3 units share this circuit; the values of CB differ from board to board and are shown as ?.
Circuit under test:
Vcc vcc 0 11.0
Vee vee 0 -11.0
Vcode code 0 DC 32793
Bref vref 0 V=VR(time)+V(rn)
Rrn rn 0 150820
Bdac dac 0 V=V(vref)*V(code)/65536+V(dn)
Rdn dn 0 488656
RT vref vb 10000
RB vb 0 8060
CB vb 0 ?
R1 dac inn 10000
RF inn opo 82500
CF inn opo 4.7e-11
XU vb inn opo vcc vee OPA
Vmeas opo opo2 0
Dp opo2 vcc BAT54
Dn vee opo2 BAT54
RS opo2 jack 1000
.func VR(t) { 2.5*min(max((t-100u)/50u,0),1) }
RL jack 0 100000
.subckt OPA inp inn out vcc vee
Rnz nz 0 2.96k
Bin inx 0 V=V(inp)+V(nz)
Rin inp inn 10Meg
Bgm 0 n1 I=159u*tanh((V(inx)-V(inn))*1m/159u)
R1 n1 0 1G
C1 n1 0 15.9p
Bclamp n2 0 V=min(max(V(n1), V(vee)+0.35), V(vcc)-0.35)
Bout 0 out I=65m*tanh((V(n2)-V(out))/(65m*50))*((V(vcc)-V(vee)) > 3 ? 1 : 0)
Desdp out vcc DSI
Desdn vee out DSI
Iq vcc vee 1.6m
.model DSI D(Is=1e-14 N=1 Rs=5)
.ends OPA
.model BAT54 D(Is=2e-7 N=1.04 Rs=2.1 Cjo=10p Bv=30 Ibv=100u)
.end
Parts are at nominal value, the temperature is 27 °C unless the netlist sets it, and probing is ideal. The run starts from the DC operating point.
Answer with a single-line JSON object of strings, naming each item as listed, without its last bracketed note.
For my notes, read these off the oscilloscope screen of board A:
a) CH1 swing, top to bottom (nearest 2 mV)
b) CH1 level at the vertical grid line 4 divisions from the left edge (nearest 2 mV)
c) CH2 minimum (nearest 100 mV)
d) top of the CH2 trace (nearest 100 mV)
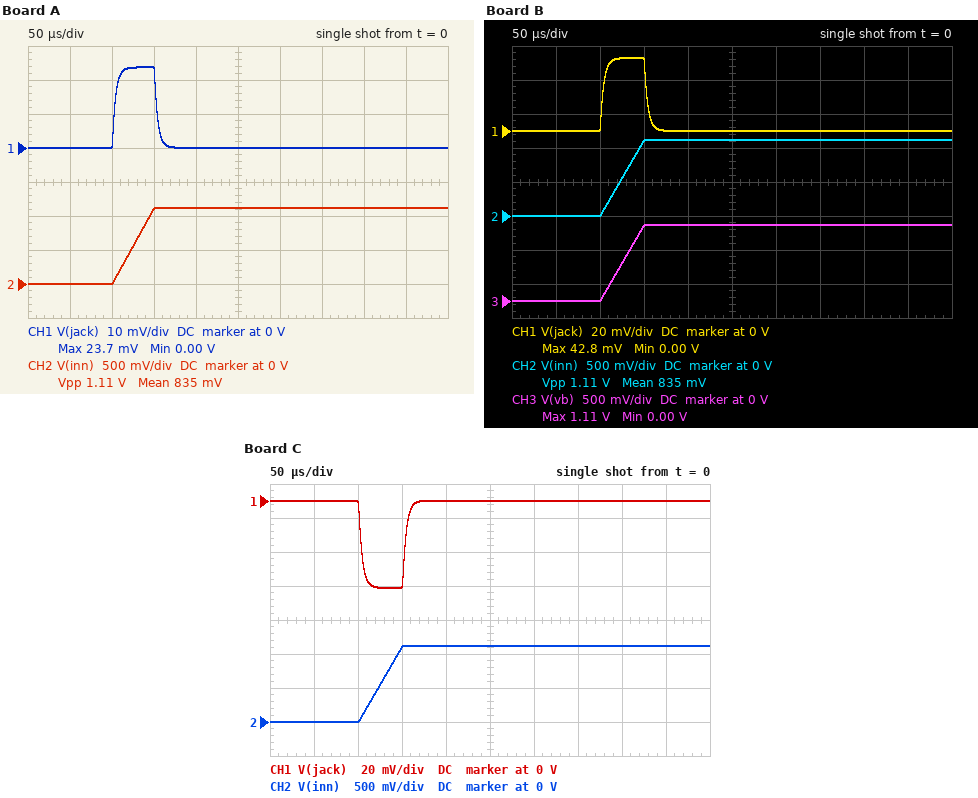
{"CH1 swing, top to bottom": "24 mV", "CH1 level at the vertical grid line 4 divisions from the left edge": "0 V", "CH2 minimum": "0 V", "top of the CH2 trace": "1.1 V"}
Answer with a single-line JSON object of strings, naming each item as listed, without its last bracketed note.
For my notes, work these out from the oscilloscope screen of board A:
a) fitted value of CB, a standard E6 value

{"fitted value of CB, a standard E6 value": "68 pF"}
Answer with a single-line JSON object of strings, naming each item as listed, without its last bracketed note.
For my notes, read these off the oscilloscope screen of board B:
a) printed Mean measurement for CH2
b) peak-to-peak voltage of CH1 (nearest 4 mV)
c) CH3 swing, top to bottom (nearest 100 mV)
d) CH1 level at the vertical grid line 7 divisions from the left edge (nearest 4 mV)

{"printed Mean measurement for CH2": "835 mV", "peak-to-peak voltage of CH1": "44 mV", "CH3 swing, top to bottom": "1.1 V", "CH1 level at the vertical grid line 7 divisions from the left edge": "0 V"}
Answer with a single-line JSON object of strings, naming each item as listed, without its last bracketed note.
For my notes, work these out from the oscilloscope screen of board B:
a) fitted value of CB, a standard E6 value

{"fitted value of CB, a standard E6 value": "47 pF"}
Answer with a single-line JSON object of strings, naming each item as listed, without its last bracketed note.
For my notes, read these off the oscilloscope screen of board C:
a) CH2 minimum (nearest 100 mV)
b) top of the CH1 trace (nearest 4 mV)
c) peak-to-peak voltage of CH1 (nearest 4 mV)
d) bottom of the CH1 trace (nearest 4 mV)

{"CH2 minimum": "0 V", "top of the CH1 trace": "0 V", "peak-to-peak voltage of CH1": "52 mV", "bottom of the CH1 trace": "-52 mV"}
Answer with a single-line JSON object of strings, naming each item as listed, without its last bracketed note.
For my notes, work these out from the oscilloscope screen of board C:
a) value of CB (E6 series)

{"value of CB": "150 pF"}
